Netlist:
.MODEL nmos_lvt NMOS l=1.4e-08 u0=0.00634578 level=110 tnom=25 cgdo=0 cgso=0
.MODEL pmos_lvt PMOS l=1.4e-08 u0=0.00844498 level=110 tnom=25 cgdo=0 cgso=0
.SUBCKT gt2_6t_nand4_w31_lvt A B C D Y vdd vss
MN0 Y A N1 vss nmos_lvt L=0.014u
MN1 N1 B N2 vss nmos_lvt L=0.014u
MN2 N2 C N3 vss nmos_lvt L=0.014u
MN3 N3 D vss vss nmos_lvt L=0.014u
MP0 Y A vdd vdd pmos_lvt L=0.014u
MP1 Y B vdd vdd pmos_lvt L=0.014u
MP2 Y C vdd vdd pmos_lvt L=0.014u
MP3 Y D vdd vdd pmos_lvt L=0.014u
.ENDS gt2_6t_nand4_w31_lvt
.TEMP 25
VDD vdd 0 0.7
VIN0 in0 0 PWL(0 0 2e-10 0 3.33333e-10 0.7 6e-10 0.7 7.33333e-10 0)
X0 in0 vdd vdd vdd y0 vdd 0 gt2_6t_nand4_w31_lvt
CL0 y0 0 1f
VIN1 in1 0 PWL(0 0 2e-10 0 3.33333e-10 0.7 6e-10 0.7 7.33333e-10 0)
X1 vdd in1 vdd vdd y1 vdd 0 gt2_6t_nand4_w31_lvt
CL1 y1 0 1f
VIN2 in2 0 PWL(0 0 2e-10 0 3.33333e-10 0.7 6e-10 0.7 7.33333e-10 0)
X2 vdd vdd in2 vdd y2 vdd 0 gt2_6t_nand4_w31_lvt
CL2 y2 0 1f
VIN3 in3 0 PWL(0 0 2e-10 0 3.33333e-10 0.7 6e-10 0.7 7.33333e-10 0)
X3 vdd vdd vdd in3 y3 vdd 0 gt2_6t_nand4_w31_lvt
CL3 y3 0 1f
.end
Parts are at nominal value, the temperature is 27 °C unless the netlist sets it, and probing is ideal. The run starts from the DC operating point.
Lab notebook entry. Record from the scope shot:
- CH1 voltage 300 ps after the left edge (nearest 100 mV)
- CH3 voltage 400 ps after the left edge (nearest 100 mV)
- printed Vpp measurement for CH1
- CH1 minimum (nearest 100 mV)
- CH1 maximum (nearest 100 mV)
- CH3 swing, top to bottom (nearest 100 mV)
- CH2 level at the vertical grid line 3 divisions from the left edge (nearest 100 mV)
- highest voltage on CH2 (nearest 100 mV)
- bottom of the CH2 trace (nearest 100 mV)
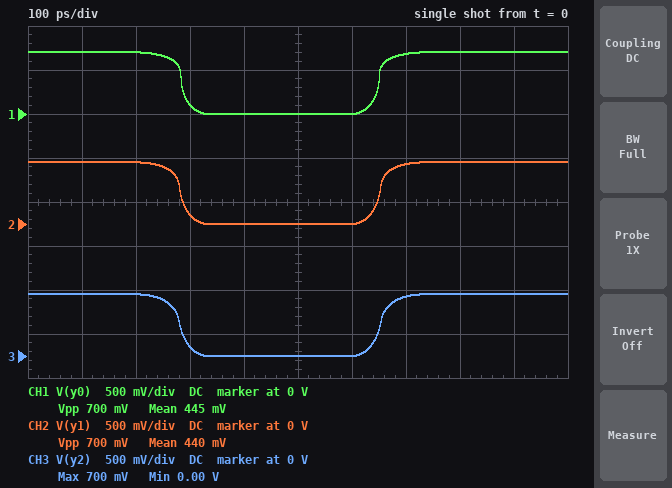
100 mV
0 V
700 mV
0 V
700 mV
700 mV
100 mV
700 mV
0 V
